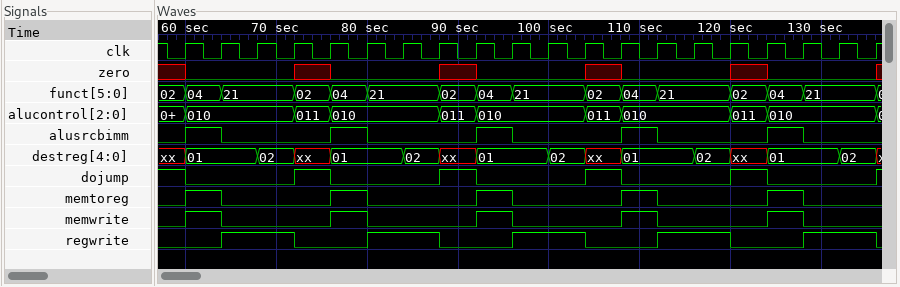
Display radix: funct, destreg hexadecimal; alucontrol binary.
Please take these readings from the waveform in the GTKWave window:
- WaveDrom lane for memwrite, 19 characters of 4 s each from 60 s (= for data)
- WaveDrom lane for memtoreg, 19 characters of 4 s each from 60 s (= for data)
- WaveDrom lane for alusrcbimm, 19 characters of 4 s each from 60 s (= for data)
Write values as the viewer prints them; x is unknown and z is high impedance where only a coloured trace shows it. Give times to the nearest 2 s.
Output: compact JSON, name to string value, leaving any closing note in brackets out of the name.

{"WaveDrom lane for memwrite, 19 characters of 4 s each from 60 s": "{name: 'memwrite', wave: '10..10..10..10..10.'}", "WaveDrom lane for memtoreg, 19 characters of 4 s each from 60 s": "{name: 'memtoreg', wave: '10..10..10..10..10.'}", "WaveDrom lane for alusrcbimm, 19 characters of 4 s each from 60 s": "{name: 'alusrcbimm', wave: '10..10..10..10..10.'}"}
